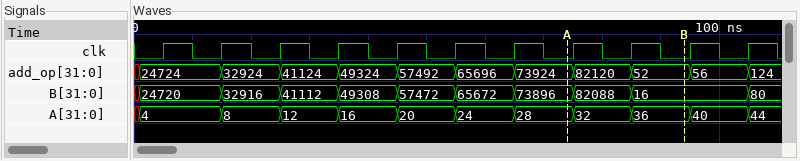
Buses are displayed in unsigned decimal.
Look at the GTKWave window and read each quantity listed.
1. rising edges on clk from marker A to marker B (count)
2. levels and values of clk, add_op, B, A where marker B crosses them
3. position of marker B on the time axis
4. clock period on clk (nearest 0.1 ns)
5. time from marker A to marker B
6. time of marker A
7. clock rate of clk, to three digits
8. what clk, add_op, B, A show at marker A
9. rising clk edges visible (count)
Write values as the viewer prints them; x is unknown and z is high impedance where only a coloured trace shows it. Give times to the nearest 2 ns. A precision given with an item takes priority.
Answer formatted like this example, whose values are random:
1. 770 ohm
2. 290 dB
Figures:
1. 2
2. clk=0, add_op=52, B=16, A=36
3. 94 ns
4. 10 ns
5. 20 ns
6. 74 ns
7. 100 MHz
8. clk=0, add_op=73924, B=73896, A=28
9. 11
